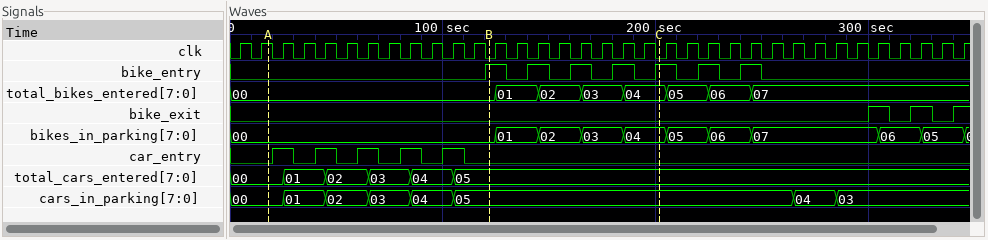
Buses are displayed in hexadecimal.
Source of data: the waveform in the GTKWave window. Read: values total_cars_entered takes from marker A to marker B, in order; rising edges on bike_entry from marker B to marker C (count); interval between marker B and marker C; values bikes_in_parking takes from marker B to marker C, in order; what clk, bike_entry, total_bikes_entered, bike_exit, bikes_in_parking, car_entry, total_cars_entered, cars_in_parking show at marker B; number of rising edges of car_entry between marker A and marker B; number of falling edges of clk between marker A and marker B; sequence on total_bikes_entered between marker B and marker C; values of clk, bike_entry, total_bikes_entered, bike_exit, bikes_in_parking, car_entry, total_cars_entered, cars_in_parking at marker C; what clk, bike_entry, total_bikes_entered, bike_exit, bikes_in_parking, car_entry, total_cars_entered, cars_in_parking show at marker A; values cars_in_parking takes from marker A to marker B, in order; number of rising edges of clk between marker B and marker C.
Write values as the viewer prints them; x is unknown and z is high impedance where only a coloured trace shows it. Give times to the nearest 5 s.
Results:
00, 01, 02, 03, 04, 05
4
80 s
00, 01, 02, 03, 04
clk=0, bike_entry=1, total_bikes_entered=00, bike_exit=0, bikes_in_parking=00, car_entry=0, total_cars_entered=05, cars_in_parking=05
5
11
00, 01, 02, 03, 04
clk=0, bike_entry=1, total_bikes_entered=04, bike_exit=0, bikes_in_parking=04, car_entry=0, total_cars_entered=05, cars_in_parking=05
clk=1, bike_entry=0, total_bikes_entered=00, bike_exit=0, bikes_in_parking=00, car_entry=0, total_cars_entered=00, cars_in_parking=00
00, 01, 02, 03, 04, 05
8
